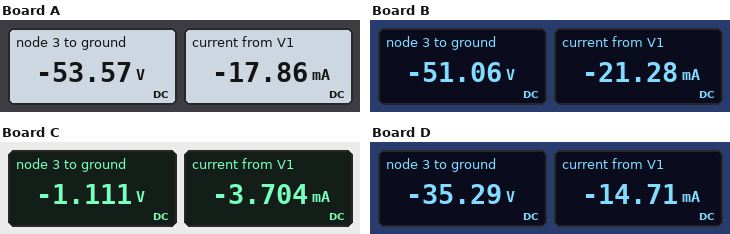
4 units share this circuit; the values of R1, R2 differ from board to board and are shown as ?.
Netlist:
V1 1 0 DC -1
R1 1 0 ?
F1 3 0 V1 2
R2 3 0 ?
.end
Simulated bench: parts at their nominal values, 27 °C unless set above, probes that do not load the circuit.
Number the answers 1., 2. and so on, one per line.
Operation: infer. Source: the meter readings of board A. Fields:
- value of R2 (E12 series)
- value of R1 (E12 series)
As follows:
1. 1.5 kΩ
2. 56 Ω
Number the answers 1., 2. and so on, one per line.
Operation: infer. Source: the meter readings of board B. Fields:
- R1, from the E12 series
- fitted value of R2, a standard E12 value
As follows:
1. 47 Ω
2. 1.2 kΩ
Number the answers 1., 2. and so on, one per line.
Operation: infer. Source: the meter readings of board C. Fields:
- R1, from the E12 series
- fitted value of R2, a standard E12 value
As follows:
1. 270 Ω
2. 150 Ω
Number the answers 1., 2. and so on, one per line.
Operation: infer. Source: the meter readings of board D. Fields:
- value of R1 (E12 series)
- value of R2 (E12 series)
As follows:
1. 68 Ω
2. 1.2 kΩ
